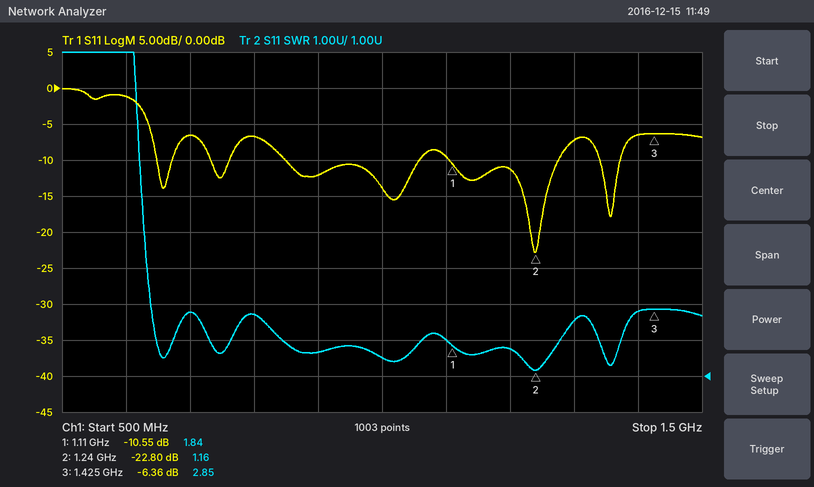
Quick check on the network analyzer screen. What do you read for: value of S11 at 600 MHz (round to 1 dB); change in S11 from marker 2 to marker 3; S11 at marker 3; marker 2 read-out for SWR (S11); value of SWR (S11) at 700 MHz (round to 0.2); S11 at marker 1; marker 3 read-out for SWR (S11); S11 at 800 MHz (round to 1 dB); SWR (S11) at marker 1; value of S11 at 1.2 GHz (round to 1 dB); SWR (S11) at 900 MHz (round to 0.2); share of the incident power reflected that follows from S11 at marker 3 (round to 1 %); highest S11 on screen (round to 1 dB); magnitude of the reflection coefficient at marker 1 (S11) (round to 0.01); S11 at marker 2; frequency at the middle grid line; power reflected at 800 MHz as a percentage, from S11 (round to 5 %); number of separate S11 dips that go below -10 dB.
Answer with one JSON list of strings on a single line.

["-1 dB", "16.44 dB", "-6.36 dB", "1.16", "2.8", "-10.55 dB", "2.85", "-7 dB", "1.84", "-11 dB", "1.6", "23 %", "0 dB", "0.30", "-22.80 dB", "1 GHz", "20 %", "5"]
